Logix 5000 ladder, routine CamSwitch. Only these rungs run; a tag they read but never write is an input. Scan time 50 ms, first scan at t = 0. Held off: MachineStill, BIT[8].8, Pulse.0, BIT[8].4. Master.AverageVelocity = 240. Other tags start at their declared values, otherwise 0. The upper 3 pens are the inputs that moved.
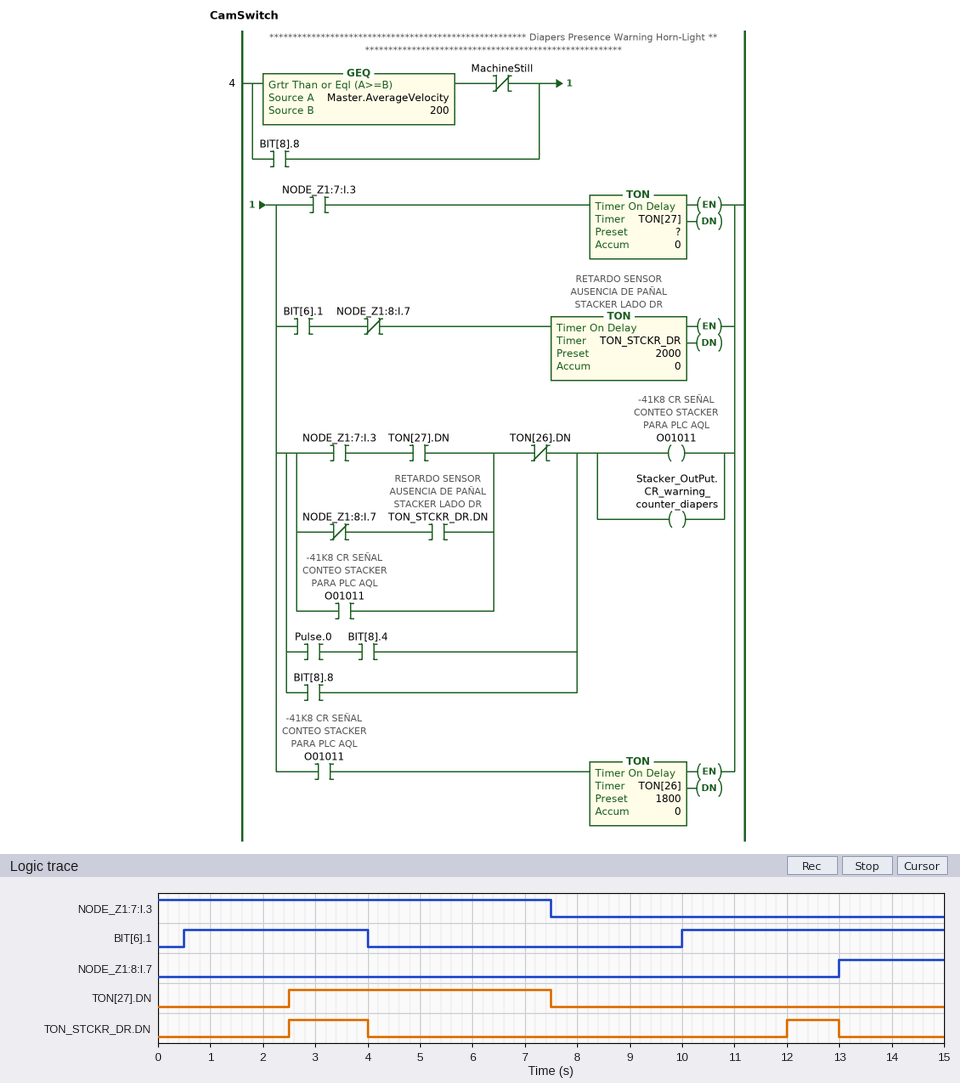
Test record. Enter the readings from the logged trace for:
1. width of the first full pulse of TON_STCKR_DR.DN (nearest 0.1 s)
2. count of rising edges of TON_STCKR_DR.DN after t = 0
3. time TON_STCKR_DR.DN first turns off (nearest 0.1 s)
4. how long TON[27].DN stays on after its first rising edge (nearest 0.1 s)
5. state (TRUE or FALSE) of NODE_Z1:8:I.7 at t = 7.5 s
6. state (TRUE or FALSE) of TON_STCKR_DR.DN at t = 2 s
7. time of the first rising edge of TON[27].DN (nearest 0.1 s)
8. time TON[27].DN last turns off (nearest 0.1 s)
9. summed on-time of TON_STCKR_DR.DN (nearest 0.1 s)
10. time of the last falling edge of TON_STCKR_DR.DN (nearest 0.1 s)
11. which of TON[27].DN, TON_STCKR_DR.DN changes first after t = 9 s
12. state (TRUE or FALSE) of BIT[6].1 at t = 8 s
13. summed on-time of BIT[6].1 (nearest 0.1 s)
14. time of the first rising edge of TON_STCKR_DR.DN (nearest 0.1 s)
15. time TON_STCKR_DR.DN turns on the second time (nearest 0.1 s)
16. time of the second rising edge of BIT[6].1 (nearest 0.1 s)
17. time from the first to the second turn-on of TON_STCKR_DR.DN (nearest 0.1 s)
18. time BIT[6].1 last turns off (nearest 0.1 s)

1.5 s
2
4.0 s
5.0 s
FALSE
FALSE
2.5 s
7.5 s
2.5 s
13.0 s
TON_STCKR_DR.DN
FALSE
8.5 s
2.5 s
12.0 s
10.0 s
9.5 s
4.0 s
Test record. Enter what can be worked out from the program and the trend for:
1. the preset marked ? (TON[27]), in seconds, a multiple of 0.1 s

2.5 s
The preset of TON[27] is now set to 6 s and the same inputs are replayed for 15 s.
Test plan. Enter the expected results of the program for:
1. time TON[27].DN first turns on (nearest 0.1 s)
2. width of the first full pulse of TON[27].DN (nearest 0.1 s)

6.0 s
1.5 s
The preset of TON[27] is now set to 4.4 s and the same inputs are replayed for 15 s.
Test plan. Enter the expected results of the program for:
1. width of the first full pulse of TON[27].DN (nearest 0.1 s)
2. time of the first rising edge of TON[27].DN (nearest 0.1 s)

3.1 s
4.4 s
